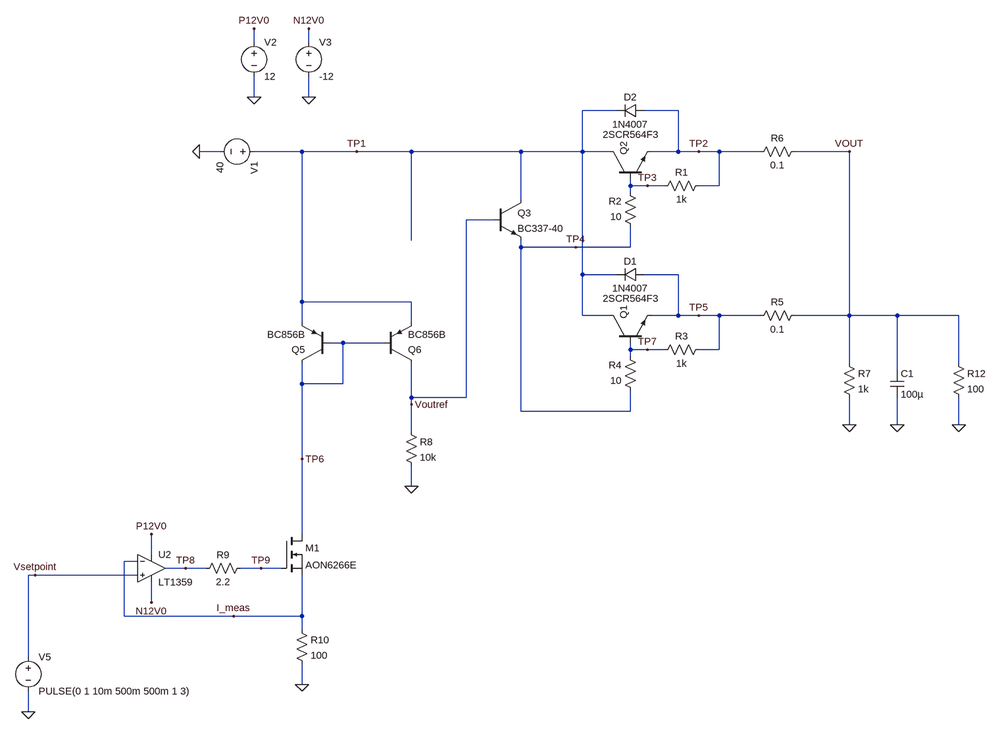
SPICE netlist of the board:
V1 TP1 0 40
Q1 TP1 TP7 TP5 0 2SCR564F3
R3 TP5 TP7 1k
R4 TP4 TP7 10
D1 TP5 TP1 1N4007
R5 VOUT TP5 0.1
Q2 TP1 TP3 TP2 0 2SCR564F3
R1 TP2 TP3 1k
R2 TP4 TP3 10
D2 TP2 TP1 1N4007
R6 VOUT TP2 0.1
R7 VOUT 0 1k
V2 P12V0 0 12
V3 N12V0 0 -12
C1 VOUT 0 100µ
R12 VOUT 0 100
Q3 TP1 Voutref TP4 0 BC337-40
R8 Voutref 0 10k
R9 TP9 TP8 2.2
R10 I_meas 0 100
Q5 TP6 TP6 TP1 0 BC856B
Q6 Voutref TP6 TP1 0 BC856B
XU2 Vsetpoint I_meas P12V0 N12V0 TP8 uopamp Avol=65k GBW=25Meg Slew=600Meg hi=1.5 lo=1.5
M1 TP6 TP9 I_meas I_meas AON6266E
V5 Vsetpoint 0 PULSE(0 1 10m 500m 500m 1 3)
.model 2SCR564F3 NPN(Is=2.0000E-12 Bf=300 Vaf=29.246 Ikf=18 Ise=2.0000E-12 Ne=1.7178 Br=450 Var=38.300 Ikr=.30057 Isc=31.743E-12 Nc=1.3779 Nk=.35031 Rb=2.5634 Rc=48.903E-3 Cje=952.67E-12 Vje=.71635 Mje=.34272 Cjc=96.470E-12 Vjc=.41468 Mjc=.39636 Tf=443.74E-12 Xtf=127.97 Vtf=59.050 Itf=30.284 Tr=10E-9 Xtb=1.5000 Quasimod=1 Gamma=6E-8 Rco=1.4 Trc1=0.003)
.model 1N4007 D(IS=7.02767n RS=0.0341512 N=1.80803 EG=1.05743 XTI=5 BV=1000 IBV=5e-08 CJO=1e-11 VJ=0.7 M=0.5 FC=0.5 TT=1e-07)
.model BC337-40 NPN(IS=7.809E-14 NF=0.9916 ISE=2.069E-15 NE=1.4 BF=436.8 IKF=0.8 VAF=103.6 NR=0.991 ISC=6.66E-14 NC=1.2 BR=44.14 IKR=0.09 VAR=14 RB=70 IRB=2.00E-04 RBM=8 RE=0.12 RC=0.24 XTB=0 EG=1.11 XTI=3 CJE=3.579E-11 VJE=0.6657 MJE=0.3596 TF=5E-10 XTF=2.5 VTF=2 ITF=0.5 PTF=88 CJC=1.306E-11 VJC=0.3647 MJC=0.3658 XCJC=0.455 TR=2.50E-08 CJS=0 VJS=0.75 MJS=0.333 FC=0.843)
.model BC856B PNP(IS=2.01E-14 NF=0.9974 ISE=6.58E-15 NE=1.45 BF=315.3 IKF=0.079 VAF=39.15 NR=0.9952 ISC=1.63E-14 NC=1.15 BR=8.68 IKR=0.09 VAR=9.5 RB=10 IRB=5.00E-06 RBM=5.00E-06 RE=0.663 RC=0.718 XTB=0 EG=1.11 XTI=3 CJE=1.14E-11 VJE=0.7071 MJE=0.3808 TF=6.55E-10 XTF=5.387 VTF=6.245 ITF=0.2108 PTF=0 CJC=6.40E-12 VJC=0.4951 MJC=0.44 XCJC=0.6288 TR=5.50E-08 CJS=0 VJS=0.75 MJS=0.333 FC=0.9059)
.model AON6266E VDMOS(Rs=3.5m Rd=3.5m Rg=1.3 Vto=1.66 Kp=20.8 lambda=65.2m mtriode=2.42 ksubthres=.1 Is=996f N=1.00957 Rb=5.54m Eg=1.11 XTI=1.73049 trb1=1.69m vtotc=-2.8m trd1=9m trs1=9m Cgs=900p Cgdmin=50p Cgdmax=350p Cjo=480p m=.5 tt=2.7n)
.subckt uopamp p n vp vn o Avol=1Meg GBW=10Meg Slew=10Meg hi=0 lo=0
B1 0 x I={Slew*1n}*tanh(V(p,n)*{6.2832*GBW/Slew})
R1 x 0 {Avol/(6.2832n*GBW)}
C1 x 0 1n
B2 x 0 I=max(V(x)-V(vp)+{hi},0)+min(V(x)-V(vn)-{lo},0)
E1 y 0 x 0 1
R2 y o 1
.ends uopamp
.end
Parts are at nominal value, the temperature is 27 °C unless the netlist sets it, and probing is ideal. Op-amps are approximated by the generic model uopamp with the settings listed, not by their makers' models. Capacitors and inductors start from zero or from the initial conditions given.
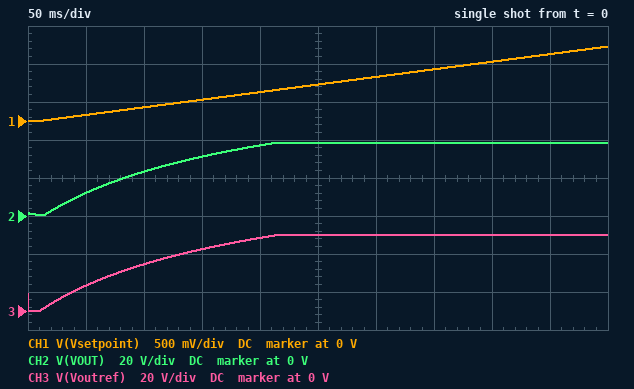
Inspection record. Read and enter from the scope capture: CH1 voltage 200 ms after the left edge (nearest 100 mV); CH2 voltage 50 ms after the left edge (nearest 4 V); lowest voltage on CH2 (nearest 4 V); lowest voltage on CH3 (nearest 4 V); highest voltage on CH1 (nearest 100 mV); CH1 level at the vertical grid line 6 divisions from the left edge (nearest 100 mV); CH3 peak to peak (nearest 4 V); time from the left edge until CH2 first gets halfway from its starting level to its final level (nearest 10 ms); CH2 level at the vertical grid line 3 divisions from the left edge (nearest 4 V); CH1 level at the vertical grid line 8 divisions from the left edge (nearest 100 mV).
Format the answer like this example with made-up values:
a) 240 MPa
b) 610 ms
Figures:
a) 400 mV
b) 12 V
c) 0 V
d) 0 V
e) 1.0 V
f) 600 mV
g) 40 V
h) 80 ms
i) 32 V
j) 800 mV
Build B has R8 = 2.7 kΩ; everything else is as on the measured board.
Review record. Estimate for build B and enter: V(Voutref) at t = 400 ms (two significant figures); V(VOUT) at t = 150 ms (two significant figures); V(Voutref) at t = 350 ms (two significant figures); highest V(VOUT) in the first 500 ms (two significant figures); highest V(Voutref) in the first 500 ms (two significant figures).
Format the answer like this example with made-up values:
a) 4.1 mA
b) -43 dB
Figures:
a) 27 V
b) 11 V
c) 24 V
d) 30 V
e) 31 V
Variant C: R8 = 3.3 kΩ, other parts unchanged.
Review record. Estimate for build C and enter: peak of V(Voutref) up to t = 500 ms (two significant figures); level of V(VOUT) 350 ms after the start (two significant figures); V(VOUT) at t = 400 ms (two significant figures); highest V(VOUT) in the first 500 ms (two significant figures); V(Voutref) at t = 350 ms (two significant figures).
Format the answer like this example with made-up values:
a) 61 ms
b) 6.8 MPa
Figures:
a) 35 V
b) 27 V
c) 29 V
d) 34 V
e) 28 V
